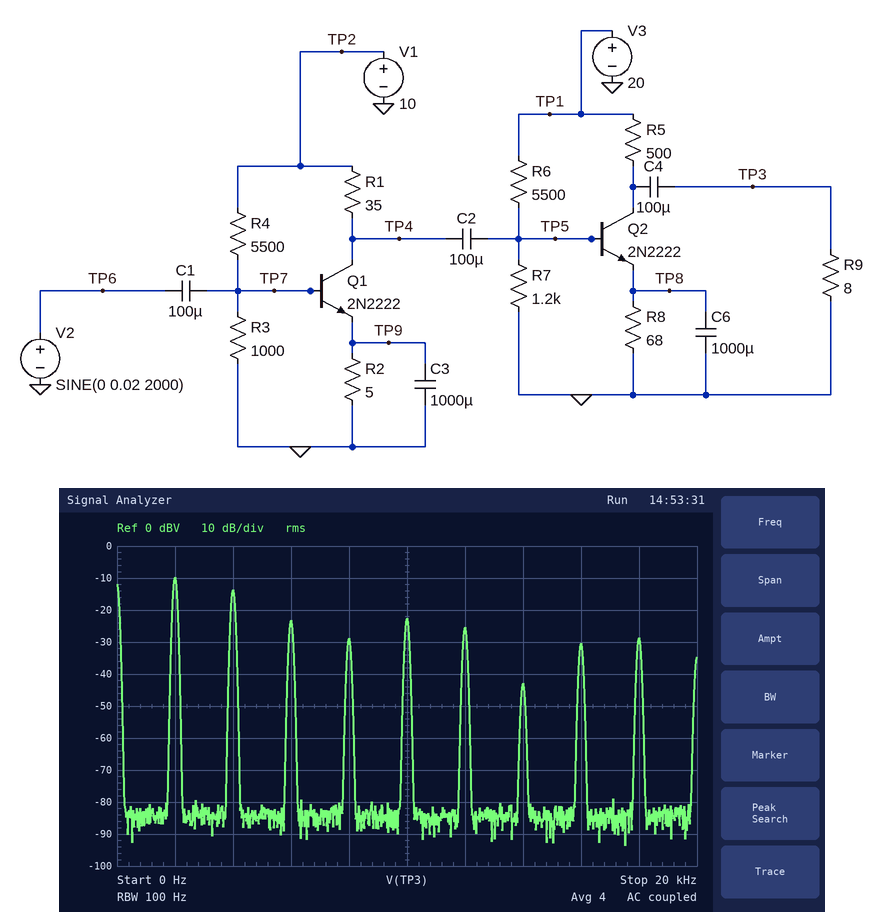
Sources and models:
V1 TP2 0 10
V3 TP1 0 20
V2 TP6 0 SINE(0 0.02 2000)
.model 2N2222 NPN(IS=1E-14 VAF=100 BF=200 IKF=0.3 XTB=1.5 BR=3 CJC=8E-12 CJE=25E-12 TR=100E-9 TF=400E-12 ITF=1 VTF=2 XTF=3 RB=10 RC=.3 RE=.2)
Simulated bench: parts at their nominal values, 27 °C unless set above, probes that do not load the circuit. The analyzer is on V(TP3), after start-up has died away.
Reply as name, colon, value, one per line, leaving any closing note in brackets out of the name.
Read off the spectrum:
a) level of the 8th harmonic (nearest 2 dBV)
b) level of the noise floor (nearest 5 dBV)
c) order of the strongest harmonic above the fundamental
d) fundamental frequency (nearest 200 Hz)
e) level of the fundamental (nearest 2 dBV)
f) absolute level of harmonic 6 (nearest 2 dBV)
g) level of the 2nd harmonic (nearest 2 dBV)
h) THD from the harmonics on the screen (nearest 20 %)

level of the 8th harmonic: -30 dBV
level of the noise floor: -85 dBV
order of the strongest harmonic above the fundamental: 2
fundamental frequency: 2.0 kHz
level of the fundamental: -10 dBV
absolute level of harmonic 6: -26 dBV
level of the 2nd harmonic: -14 dBV
THD from the harmonics on the screen: 80 %
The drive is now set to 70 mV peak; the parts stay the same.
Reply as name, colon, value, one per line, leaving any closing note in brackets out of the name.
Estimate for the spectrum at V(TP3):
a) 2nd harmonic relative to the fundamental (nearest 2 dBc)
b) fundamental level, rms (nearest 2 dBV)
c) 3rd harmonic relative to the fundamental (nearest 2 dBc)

2nd harmonic relative to the fundamental: -6 dBc
fundamental level, rms: -10 dBV
3rd harmonic relative to the fundamental: -24 dBc
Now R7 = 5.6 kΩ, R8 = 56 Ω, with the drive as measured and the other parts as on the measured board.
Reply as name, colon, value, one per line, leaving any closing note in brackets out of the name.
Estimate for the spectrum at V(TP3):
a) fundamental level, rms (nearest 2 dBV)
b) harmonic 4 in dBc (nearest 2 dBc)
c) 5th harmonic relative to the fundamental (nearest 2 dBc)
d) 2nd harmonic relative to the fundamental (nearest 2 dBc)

fundamental level, rms: -10 dBV
harmonic 4 in dBc: -12 dBc
5th harmonic relative to the fundamental: -24 dBc
2nd harmonic relative to the fundamental: -8 dBc
